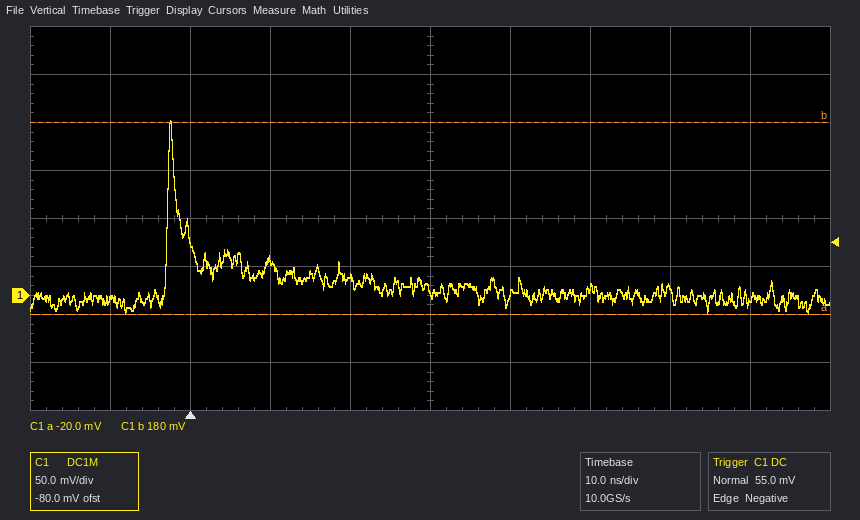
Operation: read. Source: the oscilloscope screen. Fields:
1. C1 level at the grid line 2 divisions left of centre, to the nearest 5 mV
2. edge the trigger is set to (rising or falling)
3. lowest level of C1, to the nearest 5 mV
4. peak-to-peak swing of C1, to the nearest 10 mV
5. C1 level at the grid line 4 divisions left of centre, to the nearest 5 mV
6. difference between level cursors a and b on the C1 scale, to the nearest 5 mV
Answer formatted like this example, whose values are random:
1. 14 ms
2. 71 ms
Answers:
1. 35 mV
2. falling
3. -20 mV
4. 200 mV
5. -5 mV
6. 200 mV
